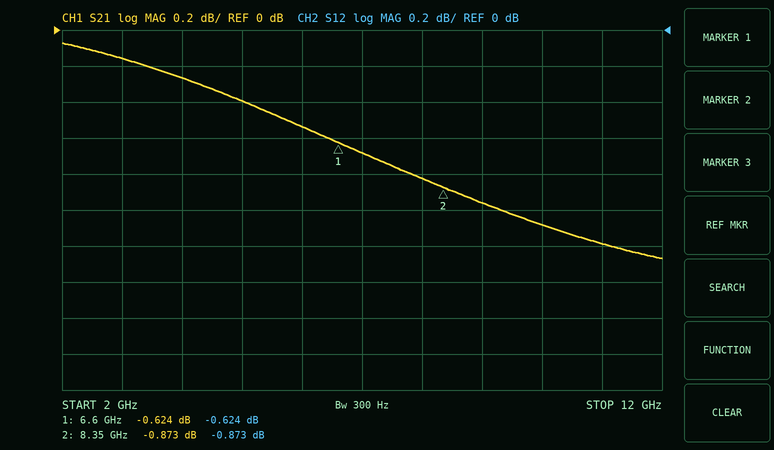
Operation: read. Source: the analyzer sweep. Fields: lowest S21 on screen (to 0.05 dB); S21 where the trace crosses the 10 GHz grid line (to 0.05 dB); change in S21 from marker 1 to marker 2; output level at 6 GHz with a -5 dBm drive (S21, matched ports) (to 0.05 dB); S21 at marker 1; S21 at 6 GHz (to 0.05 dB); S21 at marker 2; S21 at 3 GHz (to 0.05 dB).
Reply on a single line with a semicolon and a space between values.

-1.25 dB; -1.10 dB; -0.249 dB; -5.55 dBm; -0.624 dB; -0.55 dB; -0.873 dB; -0.15 dB
